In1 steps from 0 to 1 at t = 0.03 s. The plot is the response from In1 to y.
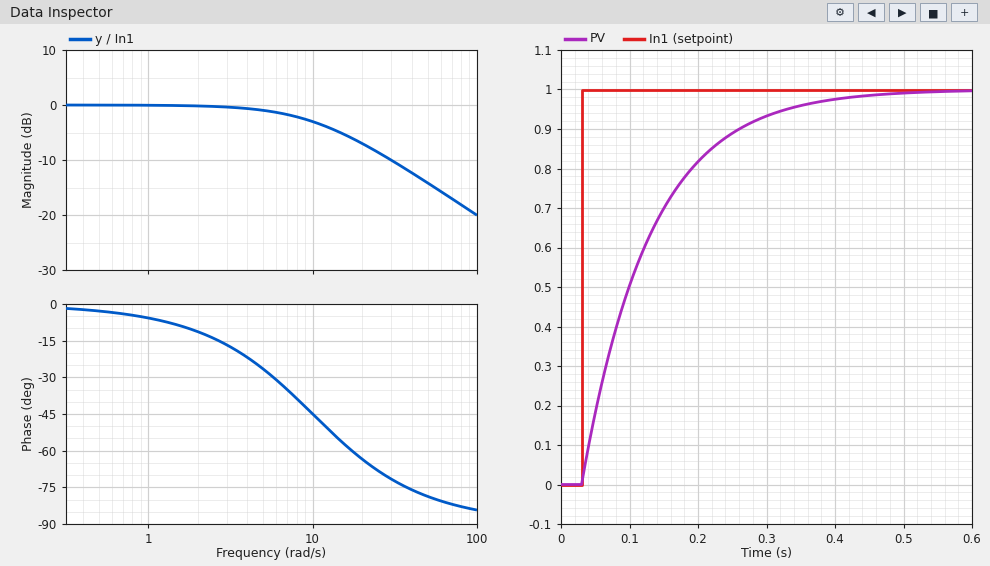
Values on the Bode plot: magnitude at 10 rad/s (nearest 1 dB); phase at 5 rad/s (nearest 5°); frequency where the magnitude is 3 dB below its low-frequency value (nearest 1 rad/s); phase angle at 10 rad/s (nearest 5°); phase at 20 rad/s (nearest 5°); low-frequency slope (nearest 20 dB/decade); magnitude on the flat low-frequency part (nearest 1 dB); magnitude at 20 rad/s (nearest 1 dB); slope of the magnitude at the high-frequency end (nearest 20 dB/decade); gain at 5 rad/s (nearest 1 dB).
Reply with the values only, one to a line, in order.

-3 dB
-25°
10 rad/s
-45°
-65°
0 dB/decade
0 dB
-7 dB
-20 dB/decade
-1 dB
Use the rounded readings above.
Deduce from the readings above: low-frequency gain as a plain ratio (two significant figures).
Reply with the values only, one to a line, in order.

1.0
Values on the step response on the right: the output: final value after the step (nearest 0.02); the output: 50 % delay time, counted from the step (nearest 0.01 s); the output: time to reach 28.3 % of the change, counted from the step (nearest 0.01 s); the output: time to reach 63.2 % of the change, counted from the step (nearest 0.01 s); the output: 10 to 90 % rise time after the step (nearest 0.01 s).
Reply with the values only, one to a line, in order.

1.00
0.07 s
0.03 s
0.10 s
0.22 s
